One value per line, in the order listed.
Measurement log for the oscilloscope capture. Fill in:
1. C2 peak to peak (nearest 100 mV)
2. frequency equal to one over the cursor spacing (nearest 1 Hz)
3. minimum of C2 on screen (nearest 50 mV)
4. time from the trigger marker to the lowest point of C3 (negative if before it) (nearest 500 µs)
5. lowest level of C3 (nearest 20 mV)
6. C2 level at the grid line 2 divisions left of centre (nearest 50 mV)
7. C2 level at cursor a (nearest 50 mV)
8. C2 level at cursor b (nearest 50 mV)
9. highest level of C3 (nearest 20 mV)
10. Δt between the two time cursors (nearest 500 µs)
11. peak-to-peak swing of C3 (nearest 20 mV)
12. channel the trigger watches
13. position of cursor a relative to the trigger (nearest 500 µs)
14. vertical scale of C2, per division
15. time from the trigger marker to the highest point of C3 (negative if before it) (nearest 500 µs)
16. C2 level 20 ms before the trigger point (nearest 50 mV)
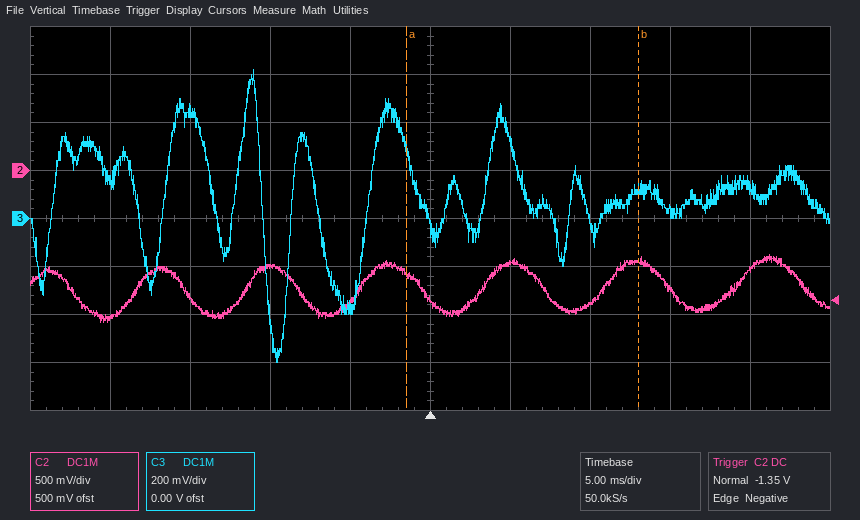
700 mV
69 Hz
-1.60 V
-9.5 ms
-600 mV
-1.00 V
-1.05 V
-950 mV
620 mV
14.5 ms
1.22 V
C2
-1.5 ms
500 mV
-11.0 ms
-1.55 V
